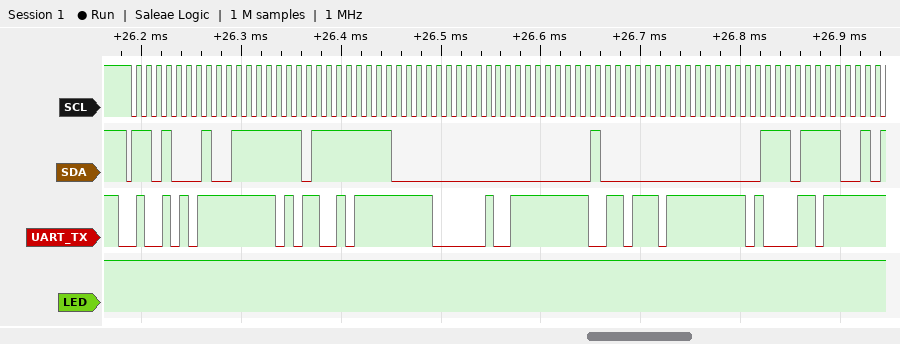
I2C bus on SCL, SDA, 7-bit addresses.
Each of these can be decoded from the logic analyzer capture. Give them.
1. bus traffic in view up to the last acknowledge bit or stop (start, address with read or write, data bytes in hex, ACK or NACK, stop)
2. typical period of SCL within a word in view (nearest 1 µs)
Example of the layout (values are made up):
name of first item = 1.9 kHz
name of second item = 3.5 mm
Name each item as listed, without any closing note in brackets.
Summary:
bus traffic in view up to the last acknowledge bit or stop = start, address 68 read ACK, 7F ACK, FF ACK, 00 ACK, 00 ACK, 40 ACK, 00 ACK, EF ACK
typical period of SCL within a word in view = 10 µs
